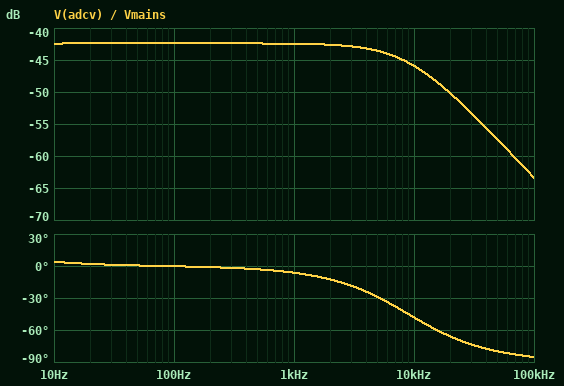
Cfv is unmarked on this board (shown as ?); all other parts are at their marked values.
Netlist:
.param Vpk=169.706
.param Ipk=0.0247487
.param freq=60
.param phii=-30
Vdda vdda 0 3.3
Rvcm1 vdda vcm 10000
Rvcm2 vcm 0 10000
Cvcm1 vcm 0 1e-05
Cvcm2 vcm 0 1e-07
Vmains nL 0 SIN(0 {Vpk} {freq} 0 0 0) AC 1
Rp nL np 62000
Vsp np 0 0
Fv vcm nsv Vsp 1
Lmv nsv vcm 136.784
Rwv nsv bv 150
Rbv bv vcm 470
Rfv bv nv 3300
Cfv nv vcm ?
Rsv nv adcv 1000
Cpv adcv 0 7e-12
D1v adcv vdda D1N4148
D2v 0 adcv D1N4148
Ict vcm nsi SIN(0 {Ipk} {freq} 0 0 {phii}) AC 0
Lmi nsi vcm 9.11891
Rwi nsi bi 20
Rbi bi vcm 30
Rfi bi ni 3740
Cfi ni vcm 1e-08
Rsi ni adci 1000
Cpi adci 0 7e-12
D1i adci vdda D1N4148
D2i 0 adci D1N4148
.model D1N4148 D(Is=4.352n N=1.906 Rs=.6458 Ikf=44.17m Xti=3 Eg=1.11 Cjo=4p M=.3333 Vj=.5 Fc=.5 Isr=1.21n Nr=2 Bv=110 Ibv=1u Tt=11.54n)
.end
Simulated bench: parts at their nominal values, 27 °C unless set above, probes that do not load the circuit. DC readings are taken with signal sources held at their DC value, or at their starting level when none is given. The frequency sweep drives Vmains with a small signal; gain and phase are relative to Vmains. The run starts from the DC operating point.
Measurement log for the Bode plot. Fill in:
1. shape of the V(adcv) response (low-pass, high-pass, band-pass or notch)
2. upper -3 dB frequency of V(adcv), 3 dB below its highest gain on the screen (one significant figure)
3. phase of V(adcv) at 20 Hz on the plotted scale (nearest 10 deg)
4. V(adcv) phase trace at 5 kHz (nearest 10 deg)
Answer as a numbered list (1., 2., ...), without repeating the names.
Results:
1. low-pass
2. 9 kHz
3. 0 deg
4. -30 deg
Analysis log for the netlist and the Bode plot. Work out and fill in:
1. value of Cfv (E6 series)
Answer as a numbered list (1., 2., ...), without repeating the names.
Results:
1. 4.7 nF
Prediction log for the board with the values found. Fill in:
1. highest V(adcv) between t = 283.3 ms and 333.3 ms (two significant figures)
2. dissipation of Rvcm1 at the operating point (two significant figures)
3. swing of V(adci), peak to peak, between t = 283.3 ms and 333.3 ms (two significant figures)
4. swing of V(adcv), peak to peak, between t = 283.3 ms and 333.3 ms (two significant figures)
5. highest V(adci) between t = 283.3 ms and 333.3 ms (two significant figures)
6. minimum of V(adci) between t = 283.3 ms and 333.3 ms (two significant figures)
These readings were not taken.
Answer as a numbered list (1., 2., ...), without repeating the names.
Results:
1. 2.9 V
2. 270 µW
3. 1.5 V
4. 2.6 V
5. 2.5 V
6. 970 mV
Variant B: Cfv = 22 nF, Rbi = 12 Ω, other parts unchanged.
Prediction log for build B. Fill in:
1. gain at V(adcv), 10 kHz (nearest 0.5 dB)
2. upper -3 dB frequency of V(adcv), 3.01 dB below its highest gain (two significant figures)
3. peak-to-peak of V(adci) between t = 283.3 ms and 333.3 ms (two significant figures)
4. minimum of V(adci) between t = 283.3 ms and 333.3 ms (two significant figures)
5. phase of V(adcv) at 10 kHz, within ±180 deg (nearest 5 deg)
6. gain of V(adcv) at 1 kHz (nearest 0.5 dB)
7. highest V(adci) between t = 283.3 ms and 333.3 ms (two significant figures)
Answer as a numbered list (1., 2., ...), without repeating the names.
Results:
1. -57.0 dB
2. 1.9 kHz
3. 600 mV
4. 1.4 V
5. -80 deg
6. -43.5 dB
7. 2.0 V
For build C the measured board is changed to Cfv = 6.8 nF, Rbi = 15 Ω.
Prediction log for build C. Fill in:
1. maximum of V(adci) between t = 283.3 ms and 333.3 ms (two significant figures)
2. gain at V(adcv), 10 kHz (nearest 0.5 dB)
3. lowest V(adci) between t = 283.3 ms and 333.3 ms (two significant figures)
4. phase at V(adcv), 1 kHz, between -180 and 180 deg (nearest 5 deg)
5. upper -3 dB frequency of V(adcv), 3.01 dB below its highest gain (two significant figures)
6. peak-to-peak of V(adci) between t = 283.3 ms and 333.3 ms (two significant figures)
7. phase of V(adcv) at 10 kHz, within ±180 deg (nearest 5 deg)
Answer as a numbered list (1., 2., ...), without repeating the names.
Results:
1. 2.1 V
2. -48.0 dB
3. 1.3 V
4. -10 deg
5. 6.2 kHz
6. 750 mV
7. -60 deg
